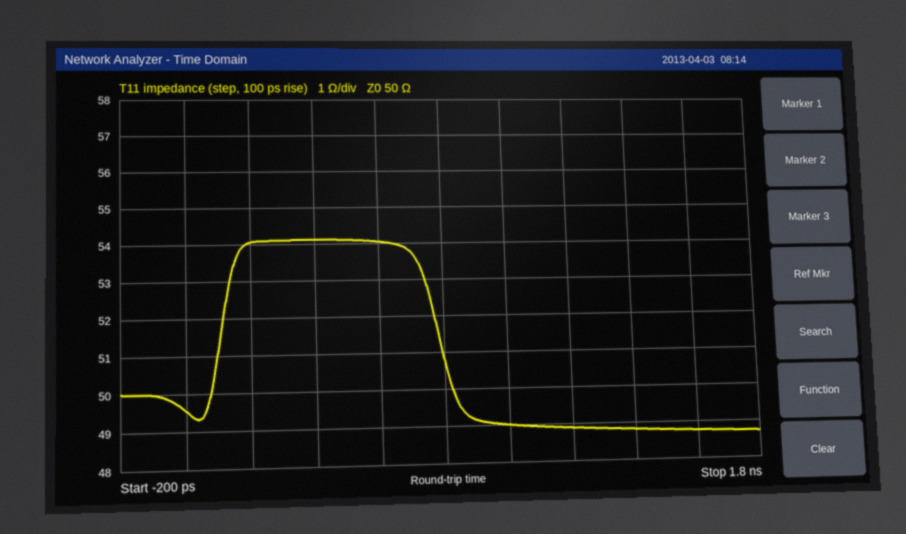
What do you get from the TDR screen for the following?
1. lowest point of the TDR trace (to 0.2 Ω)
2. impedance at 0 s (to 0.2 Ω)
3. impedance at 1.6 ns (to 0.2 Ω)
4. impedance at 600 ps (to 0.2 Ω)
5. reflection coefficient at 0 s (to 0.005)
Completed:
48.8 Ω
49.6 Ω
48.8 Ω
54.0 Ω
-0.005
